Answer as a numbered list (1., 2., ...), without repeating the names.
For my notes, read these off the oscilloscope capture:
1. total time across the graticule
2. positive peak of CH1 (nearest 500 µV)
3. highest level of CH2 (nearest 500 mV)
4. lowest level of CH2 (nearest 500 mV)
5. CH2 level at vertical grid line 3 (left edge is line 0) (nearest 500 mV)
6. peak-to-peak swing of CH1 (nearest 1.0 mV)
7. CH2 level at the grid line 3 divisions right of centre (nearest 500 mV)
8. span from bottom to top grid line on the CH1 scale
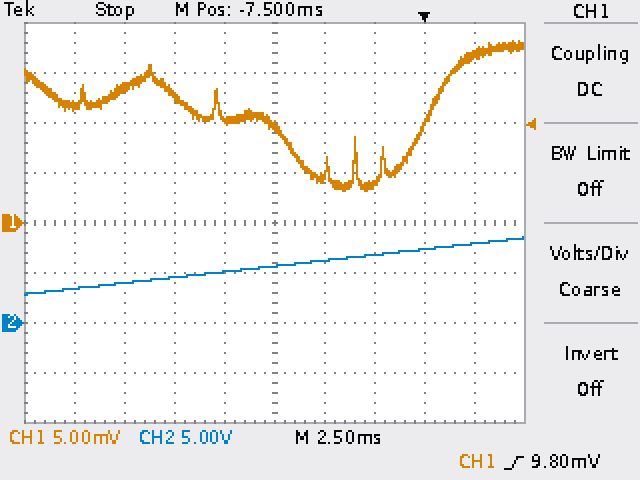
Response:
1. 25 ms
2. 18.0 mV
3. 8.5 V
4. 3.0 V
5. 4.5 V
6. 15.0 mV
7. 7.5 V
8. 40 mV
